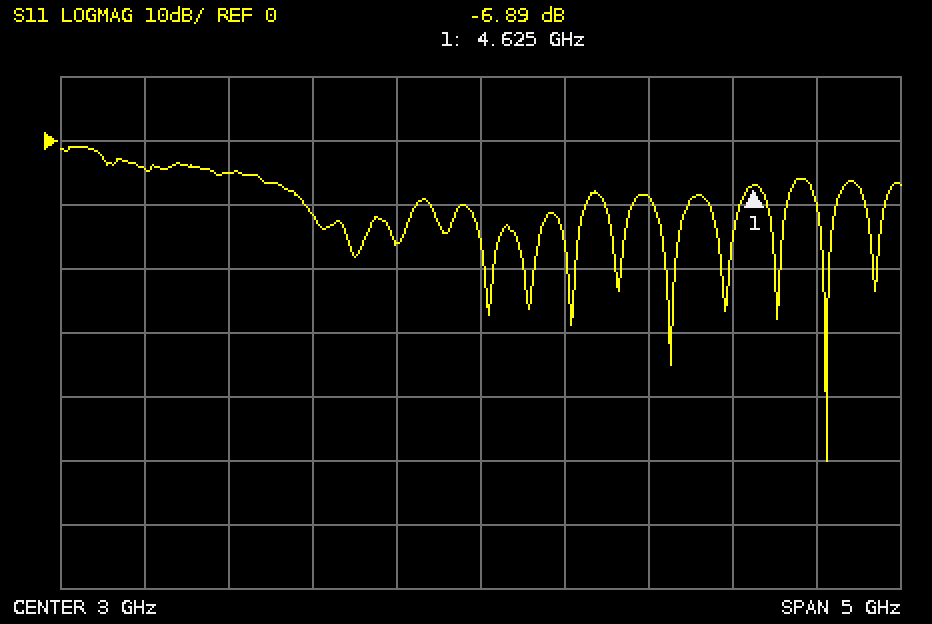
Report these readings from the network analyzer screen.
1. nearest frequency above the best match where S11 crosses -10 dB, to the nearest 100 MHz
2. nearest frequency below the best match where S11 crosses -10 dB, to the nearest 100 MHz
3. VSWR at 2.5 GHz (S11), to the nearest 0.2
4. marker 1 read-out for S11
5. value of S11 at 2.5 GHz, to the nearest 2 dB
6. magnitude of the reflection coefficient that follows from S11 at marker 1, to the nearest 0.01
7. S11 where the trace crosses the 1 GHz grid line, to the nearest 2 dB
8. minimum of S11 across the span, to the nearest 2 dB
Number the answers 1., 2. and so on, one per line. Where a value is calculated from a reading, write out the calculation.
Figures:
1. 5.1 GHz
2. 5.0 GHz
3. |Γ| = 10^(-16/20) = 0.1585; VSWR = (1 + 0.1585)/(1 − 0.1585) ≈ 1.4
4. -6.89 dB
5. -16 dB
6. 10^(-6.89/20) ≈ 0.45
7. -4 dB
8. -50 dB
